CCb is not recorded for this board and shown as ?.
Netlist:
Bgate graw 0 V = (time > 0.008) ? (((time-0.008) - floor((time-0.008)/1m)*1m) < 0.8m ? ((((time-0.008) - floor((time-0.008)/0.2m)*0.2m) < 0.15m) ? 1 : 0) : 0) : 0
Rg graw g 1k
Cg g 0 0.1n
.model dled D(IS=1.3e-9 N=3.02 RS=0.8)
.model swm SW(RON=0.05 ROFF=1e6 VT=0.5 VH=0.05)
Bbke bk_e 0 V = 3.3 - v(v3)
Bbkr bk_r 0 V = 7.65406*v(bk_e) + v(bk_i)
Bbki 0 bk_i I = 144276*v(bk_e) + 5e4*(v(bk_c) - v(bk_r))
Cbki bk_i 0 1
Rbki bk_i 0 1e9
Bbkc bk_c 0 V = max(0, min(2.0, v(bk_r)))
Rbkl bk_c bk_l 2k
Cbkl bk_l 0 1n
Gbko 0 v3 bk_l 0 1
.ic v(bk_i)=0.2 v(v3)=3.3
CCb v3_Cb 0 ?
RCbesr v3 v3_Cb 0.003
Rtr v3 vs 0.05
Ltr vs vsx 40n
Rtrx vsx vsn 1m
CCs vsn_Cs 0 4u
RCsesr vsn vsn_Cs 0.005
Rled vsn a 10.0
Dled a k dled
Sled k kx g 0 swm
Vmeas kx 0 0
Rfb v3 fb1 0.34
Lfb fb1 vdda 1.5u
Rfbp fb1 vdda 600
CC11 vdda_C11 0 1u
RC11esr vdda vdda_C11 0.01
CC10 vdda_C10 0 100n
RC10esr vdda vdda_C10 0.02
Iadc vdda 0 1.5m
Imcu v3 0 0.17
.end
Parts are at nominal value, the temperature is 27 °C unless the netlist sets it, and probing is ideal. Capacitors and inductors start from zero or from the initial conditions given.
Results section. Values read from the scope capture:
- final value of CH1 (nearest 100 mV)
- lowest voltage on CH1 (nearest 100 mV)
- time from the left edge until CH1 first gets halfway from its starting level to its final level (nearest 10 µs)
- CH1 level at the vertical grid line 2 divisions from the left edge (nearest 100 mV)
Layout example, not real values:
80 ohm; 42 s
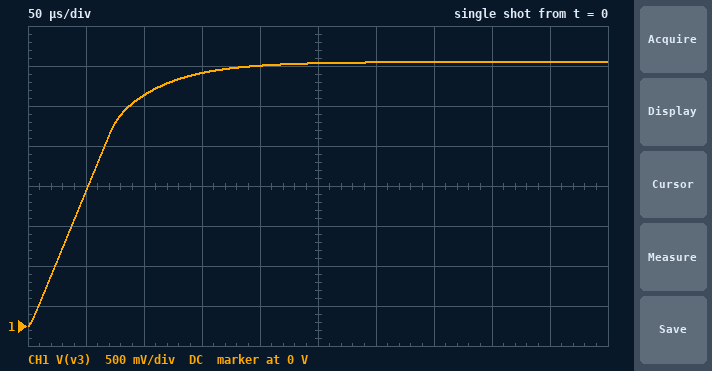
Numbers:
3.3 V; 0 V; 50 µs; 2.9 V
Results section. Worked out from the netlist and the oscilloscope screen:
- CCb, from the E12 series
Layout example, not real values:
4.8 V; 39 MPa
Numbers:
47 µF
